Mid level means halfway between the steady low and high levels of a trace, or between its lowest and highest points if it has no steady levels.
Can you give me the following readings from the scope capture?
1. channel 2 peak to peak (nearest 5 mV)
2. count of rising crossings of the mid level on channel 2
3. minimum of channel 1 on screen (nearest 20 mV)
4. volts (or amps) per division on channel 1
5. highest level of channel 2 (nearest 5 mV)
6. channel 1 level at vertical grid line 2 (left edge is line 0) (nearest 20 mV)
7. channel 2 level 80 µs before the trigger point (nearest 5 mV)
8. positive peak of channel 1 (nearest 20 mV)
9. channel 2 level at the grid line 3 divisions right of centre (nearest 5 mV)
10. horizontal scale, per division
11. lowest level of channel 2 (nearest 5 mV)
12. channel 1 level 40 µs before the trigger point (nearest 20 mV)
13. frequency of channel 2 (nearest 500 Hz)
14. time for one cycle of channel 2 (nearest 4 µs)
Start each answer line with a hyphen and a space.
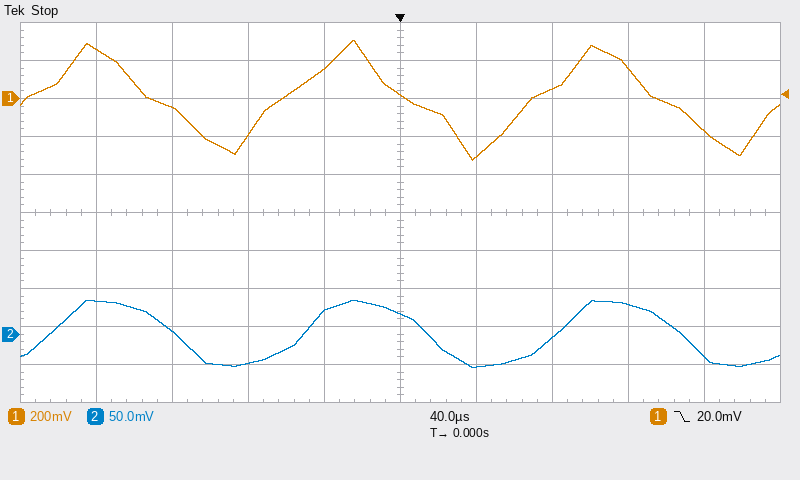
- 90 mV
- 3
- -320 mV
- 200 mV
- 45 mV
- -40 mV
- -40 mV
- 300 mV
- 40 mV
- 40 µs
- -45 mV
- 160 mV
- 7.5 kHz
- 132 µs
